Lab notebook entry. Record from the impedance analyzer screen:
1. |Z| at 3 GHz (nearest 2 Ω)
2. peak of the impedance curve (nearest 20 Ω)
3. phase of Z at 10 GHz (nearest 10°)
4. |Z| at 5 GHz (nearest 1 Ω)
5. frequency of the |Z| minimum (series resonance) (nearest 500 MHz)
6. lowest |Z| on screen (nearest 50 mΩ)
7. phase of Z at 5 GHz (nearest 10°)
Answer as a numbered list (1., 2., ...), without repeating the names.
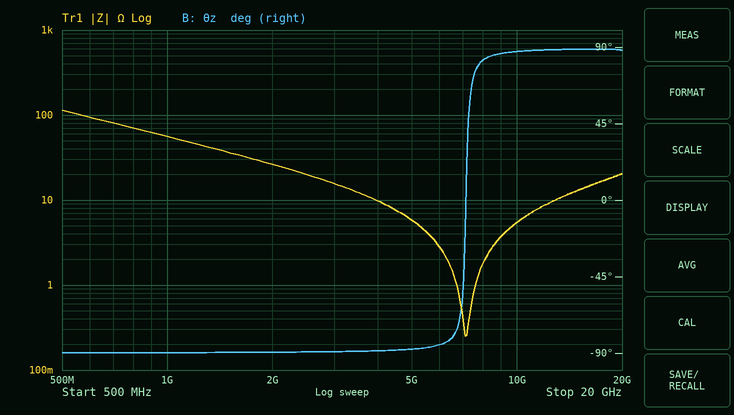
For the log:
1. 16 Ω
2. 120 Ω
3. 90°
4. 6 Ω
5. 7.0 GHz
6. 250 mΩ
7. -90°
